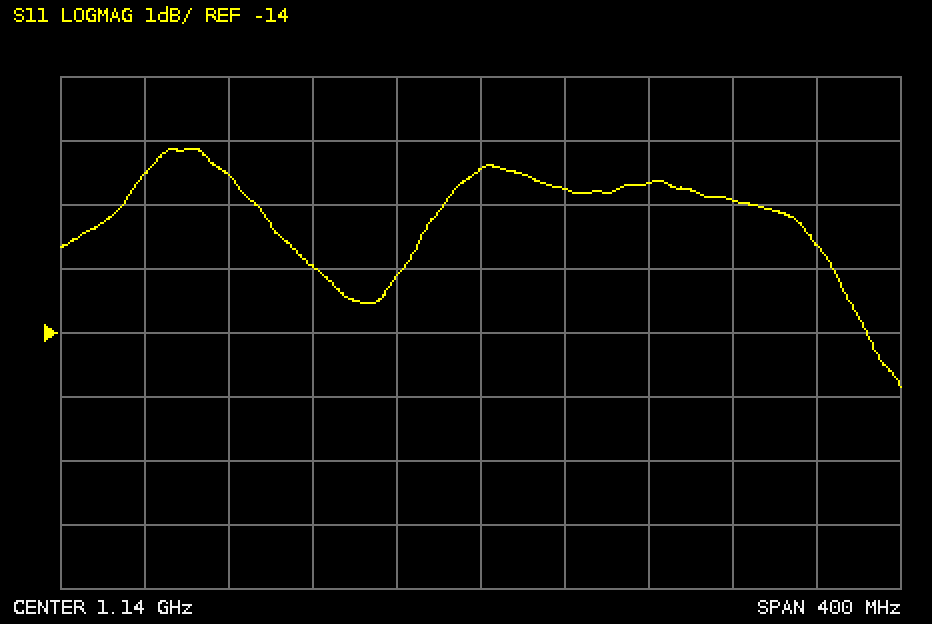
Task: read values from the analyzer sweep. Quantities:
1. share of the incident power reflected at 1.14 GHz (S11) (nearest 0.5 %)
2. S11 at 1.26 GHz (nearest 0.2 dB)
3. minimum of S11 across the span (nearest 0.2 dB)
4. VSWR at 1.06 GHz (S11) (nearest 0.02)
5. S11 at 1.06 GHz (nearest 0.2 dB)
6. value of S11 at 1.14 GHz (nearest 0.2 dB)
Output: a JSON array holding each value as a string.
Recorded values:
["7.0 %", "-12.0 dB", "-14.8 dB", "1.58", "-13.0 dB", "-11.4 dB"]
